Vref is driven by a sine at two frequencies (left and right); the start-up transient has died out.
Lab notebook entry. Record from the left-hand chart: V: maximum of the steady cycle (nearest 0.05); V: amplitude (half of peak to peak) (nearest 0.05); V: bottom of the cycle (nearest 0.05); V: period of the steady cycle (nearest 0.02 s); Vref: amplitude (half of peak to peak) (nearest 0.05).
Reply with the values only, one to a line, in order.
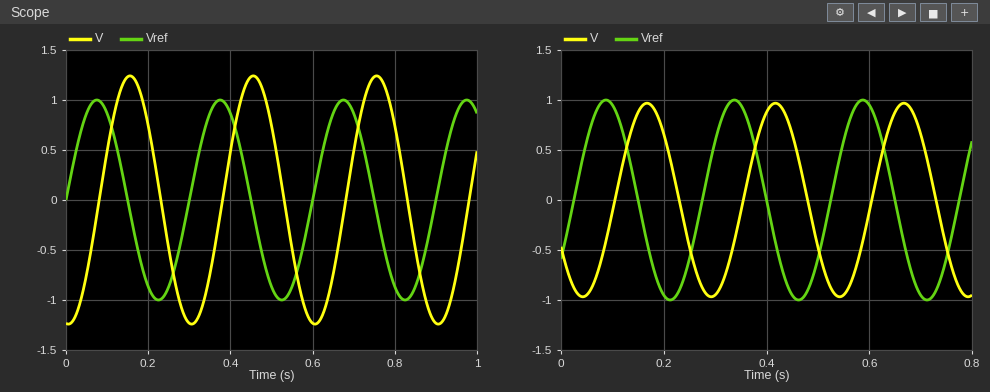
1.25
1.25
-1.25
0.30 s
1.00
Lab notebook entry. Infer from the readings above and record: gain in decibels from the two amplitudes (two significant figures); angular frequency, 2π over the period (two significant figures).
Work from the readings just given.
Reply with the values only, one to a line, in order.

1.9 dB
21 rad/s
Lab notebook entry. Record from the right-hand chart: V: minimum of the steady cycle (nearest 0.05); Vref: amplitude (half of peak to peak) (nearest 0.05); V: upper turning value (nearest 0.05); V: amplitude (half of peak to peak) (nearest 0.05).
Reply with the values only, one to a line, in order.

-0.95
1.00
0.95
0.95
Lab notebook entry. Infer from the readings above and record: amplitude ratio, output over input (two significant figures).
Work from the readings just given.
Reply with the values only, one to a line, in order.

0.95
